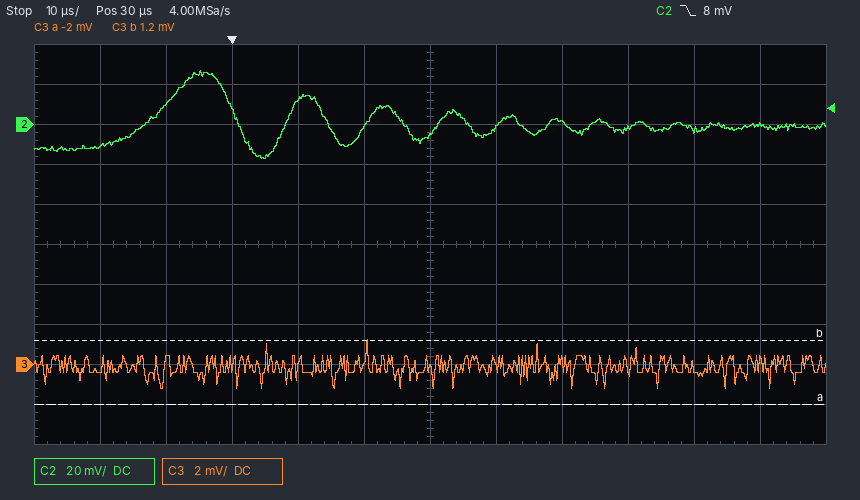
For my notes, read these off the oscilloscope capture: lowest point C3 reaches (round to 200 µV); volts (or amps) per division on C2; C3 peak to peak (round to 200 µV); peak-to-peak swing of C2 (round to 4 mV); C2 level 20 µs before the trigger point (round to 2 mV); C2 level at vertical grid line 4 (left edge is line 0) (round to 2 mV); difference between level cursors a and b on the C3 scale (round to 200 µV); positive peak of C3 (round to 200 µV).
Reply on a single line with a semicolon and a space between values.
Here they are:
-1.2 mV; 20 mV; 2.4 mV; 44 mV; -10 mV; 12 mV; 3.2 mV; 1.2 mV
